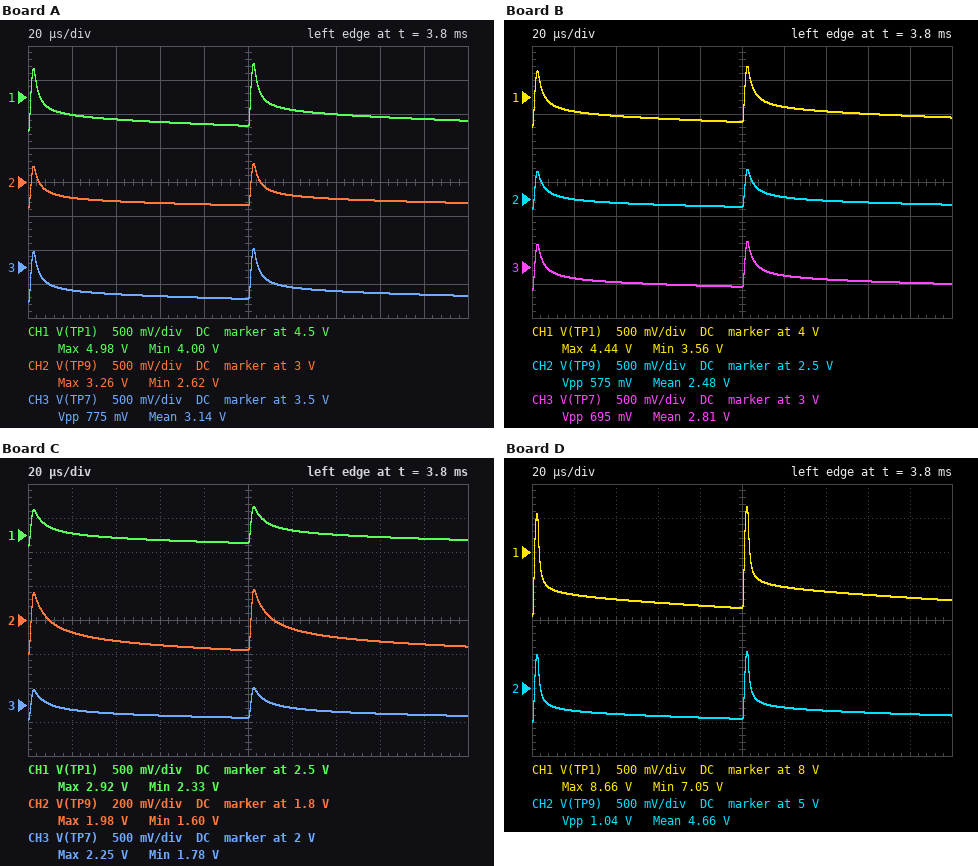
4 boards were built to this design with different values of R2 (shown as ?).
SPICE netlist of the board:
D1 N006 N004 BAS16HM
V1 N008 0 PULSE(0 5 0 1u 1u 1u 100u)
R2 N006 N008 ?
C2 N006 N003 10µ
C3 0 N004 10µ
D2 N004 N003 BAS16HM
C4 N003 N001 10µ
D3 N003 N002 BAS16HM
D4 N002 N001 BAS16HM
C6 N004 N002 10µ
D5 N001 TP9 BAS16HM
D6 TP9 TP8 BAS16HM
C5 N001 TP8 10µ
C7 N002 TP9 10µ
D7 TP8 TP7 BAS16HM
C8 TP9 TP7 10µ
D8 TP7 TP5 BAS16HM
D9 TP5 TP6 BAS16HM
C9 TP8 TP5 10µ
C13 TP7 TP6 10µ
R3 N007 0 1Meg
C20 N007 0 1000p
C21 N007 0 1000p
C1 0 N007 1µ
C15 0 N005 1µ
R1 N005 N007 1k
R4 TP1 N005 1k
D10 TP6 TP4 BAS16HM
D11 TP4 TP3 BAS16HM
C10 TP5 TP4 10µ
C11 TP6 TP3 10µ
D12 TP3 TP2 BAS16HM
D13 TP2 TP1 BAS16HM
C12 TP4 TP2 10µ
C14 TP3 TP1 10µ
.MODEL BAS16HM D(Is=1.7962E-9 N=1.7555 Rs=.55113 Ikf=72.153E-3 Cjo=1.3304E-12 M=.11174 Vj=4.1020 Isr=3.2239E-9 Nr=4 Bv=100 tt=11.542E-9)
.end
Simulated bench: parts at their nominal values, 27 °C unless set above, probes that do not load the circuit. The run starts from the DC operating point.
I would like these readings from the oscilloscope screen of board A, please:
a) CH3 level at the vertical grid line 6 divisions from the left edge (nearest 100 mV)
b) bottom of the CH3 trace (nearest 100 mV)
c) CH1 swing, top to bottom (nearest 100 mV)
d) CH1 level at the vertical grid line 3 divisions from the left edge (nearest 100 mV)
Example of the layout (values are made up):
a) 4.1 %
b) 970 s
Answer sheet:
a) 3.2 V
b) 3.0 V
c) 1.0 V
d) 4.1 V
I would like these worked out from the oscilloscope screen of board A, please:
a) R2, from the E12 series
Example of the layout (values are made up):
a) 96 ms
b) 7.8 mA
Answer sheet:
a) 1.5 Ω
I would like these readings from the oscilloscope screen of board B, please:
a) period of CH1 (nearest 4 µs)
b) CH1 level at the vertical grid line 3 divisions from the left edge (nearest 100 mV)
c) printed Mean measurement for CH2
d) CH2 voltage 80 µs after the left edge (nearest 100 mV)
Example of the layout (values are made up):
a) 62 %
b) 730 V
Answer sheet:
a) 100 µs
b) 3.7 V
c) 2.48 V
d) 2.4 V
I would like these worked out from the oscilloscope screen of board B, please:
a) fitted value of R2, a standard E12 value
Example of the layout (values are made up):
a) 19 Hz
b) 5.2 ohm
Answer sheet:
a) 1.8 Ω
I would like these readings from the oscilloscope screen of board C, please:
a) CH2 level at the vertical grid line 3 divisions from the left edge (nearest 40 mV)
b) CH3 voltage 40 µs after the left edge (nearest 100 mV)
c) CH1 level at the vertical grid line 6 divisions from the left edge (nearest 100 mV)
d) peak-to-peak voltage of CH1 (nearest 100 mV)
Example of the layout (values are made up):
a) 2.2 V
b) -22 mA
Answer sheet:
a) 1.64 V
b) 1.9 V
c) 2.6 V
d) 600 mV
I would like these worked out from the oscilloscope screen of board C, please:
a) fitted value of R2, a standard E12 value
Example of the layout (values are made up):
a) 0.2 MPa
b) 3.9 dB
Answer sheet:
a) 3.3 Ω
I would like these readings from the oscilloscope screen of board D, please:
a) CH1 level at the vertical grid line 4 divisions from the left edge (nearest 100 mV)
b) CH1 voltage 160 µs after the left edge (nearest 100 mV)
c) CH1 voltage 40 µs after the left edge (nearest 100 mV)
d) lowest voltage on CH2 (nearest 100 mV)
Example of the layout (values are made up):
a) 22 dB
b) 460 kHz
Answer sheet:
a) 7.2 V
b) 7.4 V
c) 7.3 V
d) 4.5 V
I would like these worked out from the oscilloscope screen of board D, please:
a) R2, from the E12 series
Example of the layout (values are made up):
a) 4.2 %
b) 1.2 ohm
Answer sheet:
a) 0.47 Ω
